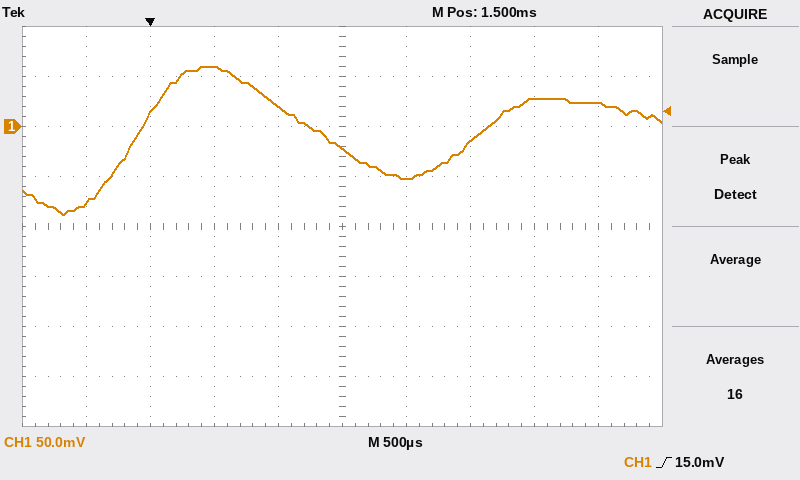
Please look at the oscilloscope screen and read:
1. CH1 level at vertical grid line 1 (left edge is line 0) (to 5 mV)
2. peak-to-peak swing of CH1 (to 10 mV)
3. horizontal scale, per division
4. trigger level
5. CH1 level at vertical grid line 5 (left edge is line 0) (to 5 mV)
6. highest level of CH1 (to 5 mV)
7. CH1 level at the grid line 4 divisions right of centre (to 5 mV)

-75 mV
150 mV
500 µs
15.0 mV
-20 mV
60 mV
25 mV
